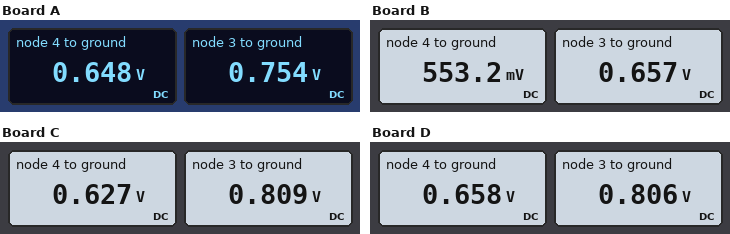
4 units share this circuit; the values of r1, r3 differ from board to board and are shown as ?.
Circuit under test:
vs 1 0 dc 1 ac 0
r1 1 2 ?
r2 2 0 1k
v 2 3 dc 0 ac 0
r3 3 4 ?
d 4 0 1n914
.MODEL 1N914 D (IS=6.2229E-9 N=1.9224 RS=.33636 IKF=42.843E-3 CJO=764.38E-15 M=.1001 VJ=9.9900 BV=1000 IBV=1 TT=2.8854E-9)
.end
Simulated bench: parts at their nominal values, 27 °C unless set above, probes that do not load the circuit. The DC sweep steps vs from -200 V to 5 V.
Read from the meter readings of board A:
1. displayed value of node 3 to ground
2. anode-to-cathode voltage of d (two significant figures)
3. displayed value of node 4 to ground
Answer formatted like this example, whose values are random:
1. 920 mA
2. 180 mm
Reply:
1. 0.754 V
2. 650 mV
3. 0.648 V
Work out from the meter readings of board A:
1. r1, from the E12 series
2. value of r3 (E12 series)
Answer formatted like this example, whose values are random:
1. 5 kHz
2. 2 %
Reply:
1. 82 Ω
2. 47 Ω
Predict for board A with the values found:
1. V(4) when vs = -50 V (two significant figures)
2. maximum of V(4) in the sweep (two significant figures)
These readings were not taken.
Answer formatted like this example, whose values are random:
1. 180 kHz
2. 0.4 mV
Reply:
1. -46 V
2. 820 mV
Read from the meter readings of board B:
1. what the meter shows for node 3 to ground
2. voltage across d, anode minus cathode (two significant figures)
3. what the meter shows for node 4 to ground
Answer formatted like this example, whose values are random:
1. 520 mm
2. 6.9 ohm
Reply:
1. 0.657 V
2. 550 mV
3. 553.2 mV
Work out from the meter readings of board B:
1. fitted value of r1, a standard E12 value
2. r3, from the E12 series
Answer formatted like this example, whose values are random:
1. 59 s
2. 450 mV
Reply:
1. 330 Ω
2. 270 Ω
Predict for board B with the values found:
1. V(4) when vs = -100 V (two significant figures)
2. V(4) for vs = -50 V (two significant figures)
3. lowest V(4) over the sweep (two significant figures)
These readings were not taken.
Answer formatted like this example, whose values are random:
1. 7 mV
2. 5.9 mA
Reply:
1. -75 V
2. -38 V
3. -150 V
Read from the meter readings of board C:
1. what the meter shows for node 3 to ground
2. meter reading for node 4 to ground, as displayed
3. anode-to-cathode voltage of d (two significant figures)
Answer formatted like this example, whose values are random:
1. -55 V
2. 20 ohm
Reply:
1. 0.809 V
2. 0.627 V
3. 630 mV
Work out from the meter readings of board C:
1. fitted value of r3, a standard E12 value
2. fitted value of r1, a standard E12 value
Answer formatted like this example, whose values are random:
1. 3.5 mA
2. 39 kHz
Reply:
1. 120 Ω
2. 82 Ω
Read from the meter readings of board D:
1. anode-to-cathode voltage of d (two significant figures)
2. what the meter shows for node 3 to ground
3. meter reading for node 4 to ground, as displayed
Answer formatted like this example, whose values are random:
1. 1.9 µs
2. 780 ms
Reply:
1. 660 mV
2. 0.806 V
3. 0.658 V
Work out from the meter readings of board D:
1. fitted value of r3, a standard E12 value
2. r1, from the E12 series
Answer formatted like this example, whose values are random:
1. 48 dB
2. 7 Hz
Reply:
1. 56 Ω
2. 56 Ω
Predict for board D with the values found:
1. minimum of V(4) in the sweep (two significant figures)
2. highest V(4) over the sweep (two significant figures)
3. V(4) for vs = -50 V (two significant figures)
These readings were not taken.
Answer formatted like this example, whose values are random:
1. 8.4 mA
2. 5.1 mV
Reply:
1. -190 V
2. 830 mV
3. -47 V
